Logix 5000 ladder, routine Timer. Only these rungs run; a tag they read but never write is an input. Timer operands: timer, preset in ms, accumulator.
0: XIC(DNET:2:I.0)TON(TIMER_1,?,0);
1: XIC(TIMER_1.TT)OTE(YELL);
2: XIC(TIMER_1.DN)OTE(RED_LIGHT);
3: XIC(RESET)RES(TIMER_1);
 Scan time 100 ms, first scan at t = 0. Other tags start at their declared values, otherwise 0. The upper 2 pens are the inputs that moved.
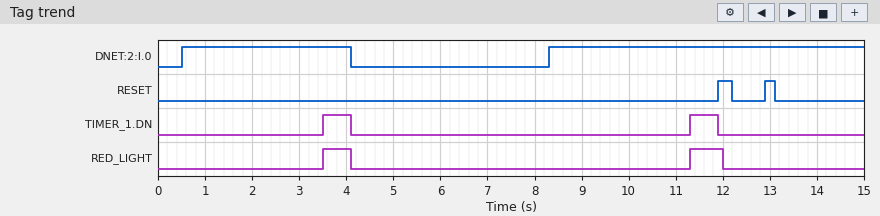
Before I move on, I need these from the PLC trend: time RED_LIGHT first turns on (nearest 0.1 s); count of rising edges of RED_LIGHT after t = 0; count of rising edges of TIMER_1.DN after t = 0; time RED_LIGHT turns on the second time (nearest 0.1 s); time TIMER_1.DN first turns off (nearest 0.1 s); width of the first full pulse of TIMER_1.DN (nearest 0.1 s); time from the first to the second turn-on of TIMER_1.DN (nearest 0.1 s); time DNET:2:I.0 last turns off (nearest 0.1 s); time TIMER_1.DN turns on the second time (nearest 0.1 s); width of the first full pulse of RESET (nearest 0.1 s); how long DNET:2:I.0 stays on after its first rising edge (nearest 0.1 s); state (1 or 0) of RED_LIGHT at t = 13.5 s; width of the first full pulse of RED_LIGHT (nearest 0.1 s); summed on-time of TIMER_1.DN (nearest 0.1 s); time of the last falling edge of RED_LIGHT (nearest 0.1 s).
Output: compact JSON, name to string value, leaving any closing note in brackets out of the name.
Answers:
{"time RED_LIGHT first turns on": "3.5 s", "count of rising edges of RED_LIGHT after t = 0": "2", "count of rising edges of TIMER_1.DN after t = 0": "2", "time RED_LIGHT turns on the second time": "11.3 s", "time TIMER_1.DN first turns off": "4.1 s", "width of the first full pulse of TIMER_1.DN": "0.6 s", "time from the first to the second turn-on of TIMER_1.DN": "7.8 s", "time DNET:2:I.0 last turns off": "4.1 s", "time TIMER_1.DN turns on the second time": "11.3 s", "width of the first full pulse of RESET": "0.3 s", "how long DNET:2:I.0 stays on after its first rising edge": "3.6 s", "state (1 or 0) of RED_LIGHT at t = 13.5 s": "0", "width of the first full pulse of RED_LIGHT": "0.6 s", "summed on-time of TIMER_1.DN": "1.2 s", "time of the last falling edge of RED_LIGHT": "12.0 s"}
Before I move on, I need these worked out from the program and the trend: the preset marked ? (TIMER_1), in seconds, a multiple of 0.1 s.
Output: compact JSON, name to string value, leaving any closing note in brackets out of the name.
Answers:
{"the preset marked ? (TIMER_1), in seconds, a multiple of 0.1 s": "3.0 s"}
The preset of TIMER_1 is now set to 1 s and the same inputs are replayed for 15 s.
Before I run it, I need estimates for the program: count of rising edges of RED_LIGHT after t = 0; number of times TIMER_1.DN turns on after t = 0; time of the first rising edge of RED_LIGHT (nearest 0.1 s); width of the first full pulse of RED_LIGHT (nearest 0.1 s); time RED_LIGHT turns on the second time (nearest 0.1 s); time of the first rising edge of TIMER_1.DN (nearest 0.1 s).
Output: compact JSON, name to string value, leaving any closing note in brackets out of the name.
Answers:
{"count of rising edges of RED_LIGHT after t = 0": "3", "number of times TIMER_1.DN turns on after t = 0": "3", "time of the first rising edge of RED_LIGHT": "1.5 s", "width of the first full pulse of RED_LIGHT": "2.6 s", "time RED_LIGHT turns on the second time": "9.3 s", "time of the first rising edge of TIMER_1.DN": "1.5 s"}
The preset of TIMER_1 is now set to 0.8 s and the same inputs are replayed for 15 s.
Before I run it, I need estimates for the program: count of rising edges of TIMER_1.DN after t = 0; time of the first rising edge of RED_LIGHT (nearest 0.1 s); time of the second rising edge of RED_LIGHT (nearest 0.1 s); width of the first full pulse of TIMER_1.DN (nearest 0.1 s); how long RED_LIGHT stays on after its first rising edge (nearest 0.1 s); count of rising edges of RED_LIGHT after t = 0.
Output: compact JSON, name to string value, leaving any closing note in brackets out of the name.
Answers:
{"count of rising edges of TIMER_1.DN after t = 0": "3", "time of the first rising edge of RED_LIGHT": "1.3 s", "time of the second rising edge of RED_LIGHT": "9.1 s", "width of the first full pulse of TIMER_1.DN": "2.8 s", "how long RED_LIGHT stays on after its first rising edge": "2.8 s", "count of rising edges of RED_LIGHT after t = 0": "3"}
